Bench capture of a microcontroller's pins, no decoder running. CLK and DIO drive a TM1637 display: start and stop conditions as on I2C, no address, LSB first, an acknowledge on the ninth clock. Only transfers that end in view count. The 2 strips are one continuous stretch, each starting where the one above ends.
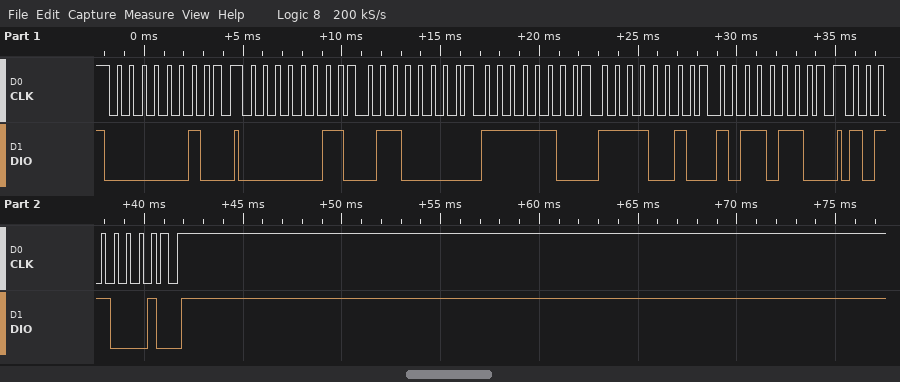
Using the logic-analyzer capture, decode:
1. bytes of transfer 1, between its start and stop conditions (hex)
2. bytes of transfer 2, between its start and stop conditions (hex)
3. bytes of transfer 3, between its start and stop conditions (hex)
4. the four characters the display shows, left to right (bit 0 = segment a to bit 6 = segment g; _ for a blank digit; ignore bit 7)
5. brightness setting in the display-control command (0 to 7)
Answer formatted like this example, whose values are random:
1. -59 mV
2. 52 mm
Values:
1. 40
2. C0 06 3F 4F 6D
3. 8D
4. 1035
5. 5
